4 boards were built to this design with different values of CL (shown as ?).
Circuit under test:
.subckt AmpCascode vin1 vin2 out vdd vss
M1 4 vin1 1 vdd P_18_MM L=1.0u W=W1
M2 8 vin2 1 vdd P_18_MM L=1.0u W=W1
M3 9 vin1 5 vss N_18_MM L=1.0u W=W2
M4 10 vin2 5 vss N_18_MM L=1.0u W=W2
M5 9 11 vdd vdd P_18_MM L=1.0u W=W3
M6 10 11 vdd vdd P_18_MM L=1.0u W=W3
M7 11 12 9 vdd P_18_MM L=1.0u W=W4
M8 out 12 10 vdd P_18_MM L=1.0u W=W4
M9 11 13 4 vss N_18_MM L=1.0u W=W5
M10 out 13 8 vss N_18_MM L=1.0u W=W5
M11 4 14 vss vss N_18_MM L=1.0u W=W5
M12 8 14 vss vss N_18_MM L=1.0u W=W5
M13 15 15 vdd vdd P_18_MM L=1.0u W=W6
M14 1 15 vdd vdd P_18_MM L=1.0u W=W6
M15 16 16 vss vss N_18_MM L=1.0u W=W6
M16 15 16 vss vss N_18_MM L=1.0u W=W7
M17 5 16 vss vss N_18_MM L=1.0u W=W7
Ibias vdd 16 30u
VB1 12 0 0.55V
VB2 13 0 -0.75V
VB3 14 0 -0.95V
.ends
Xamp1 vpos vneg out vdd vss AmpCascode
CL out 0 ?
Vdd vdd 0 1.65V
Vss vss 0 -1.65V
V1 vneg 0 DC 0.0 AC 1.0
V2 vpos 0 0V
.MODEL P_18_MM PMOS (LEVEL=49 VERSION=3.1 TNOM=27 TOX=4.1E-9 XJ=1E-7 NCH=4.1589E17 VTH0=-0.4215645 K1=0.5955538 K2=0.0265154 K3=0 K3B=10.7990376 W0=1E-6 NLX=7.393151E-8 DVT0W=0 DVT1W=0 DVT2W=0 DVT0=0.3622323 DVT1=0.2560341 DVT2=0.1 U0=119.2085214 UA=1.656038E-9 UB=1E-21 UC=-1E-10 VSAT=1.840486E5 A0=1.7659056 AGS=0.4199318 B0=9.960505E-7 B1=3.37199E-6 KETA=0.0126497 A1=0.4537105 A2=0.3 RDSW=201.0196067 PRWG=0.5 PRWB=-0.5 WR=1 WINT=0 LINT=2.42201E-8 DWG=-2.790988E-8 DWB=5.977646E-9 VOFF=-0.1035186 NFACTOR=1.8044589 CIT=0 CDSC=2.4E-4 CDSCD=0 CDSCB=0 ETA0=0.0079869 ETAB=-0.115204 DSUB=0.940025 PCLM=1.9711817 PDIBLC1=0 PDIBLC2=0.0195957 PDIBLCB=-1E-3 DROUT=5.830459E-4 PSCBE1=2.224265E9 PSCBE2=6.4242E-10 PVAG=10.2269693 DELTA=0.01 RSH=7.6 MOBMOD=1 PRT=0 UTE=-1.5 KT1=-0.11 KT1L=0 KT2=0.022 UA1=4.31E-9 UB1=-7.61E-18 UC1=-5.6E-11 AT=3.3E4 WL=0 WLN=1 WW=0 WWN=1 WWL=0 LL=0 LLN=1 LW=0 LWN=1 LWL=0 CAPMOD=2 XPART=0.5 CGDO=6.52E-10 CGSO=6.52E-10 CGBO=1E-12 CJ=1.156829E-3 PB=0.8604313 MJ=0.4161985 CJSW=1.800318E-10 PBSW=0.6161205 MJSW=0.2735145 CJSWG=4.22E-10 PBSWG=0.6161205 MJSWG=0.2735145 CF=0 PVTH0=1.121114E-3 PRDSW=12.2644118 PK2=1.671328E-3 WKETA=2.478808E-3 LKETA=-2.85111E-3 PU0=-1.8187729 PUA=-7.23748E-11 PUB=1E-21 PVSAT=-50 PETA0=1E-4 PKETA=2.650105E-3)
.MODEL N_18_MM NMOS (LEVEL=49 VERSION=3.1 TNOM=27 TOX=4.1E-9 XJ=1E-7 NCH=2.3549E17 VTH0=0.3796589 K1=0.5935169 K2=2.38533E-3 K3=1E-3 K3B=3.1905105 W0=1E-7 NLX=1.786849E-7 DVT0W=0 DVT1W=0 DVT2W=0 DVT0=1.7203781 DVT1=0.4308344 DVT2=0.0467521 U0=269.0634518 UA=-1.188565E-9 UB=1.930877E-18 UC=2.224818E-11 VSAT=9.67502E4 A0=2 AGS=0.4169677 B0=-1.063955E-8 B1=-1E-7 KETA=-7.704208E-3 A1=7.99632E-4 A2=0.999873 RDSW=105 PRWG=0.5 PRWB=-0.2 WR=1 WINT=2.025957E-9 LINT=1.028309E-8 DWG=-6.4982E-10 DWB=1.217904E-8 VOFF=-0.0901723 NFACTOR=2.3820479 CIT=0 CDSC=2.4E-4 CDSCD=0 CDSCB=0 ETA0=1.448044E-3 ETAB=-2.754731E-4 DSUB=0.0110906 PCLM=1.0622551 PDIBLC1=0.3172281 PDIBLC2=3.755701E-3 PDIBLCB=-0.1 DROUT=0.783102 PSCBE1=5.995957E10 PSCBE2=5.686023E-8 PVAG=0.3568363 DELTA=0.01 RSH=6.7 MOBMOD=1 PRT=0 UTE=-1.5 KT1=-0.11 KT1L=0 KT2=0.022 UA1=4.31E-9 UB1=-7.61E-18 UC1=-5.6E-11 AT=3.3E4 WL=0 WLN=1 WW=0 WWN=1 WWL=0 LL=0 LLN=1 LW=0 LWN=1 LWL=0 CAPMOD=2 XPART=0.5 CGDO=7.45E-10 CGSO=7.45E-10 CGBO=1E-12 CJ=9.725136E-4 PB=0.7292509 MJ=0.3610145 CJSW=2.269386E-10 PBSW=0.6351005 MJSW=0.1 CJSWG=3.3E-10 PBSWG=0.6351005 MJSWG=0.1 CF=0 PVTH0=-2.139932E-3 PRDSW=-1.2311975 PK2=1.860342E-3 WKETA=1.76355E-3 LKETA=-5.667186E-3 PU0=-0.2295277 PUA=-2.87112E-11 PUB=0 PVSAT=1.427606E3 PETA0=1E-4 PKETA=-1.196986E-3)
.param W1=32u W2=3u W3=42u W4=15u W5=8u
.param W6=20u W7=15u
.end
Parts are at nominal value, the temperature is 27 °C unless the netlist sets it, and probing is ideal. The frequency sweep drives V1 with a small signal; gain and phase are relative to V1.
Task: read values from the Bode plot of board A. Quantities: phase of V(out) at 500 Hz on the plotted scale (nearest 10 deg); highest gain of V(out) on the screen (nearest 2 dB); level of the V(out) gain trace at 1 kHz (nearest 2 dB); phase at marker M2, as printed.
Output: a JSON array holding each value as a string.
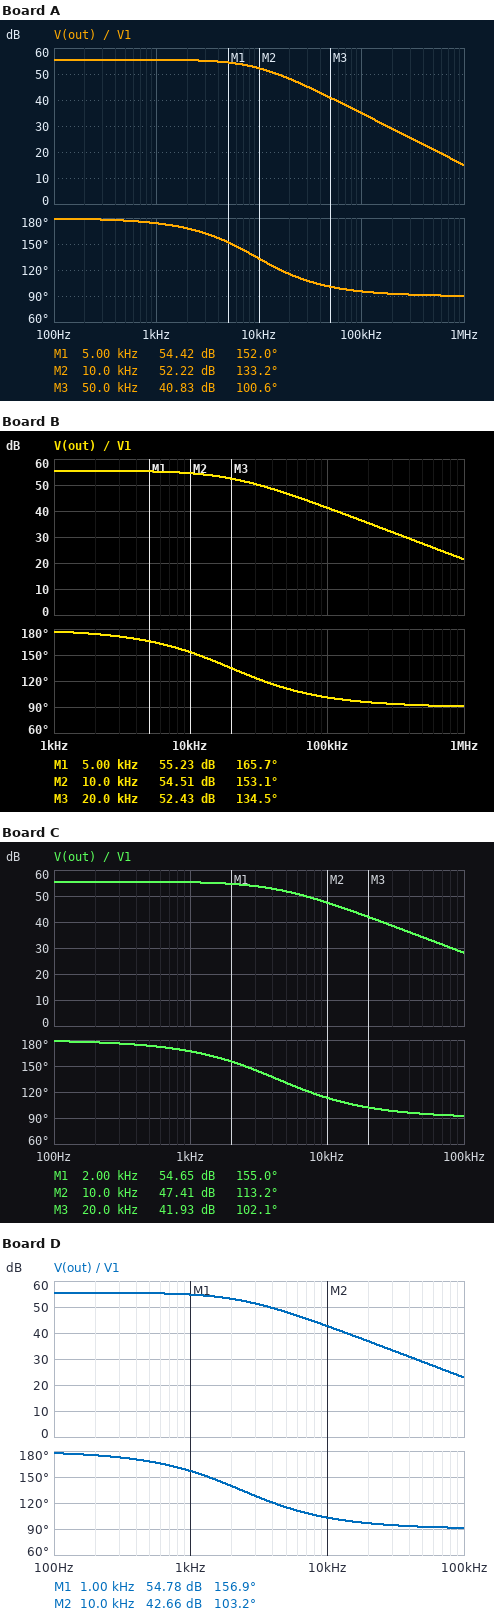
["180 deg", "56 dB", "56 dB", "133.2 deg"]
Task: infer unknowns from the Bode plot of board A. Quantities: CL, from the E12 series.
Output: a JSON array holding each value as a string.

["8.2 pF"]
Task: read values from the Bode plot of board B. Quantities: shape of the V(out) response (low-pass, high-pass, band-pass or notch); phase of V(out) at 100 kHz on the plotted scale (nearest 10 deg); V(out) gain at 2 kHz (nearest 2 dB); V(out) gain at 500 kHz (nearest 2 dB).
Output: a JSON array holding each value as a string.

["low-pass", "100 deg", "56 dB", "28 dB"]
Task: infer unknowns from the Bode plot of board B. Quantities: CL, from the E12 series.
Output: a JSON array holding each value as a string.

["3.9 pF"]
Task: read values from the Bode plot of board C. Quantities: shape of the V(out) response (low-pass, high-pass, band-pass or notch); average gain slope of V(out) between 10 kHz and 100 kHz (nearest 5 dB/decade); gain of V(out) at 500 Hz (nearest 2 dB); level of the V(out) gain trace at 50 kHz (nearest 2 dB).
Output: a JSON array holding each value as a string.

["low-pass", "-20 dB/decade", "56 dB", "34 dB"]
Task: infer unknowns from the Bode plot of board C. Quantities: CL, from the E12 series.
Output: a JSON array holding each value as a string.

["18 pF"]
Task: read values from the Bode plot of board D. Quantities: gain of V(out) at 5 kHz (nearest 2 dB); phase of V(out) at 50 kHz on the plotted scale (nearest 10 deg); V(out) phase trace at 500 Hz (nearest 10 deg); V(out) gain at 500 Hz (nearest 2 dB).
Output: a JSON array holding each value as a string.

["48 dB", "90 deg", "170 deg", "56 dB"]
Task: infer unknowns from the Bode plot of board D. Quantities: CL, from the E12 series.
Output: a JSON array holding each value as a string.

["33 pF"]
